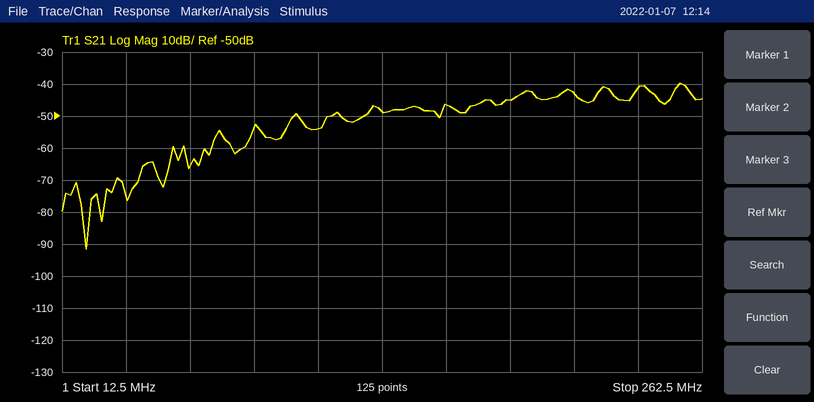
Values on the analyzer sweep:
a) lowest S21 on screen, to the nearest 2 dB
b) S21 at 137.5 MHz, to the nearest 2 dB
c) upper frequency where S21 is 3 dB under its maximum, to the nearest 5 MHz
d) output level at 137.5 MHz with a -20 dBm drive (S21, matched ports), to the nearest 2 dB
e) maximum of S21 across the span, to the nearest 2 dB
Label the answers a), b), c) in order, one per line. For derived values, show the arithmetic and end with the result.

a) -92 dB
b) -48 dB
c) 260 MHz
d) -20 dBm + (-48 dB) = -68 dBm
e) -40 dB
